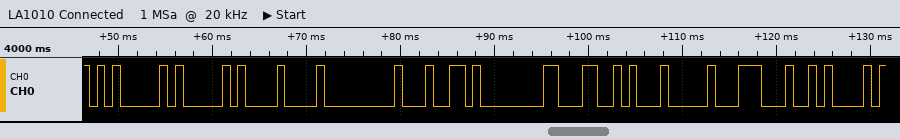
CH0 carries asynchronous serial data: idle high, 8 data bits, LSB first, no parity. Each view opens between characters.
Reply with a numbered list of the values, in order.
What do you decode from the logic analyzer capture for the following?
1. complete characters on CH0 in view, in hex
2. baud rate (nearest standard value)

1. 05, 41, 08, 00, 64, 80, 4C, 04, 1C, 0A
2. 1200 baud
